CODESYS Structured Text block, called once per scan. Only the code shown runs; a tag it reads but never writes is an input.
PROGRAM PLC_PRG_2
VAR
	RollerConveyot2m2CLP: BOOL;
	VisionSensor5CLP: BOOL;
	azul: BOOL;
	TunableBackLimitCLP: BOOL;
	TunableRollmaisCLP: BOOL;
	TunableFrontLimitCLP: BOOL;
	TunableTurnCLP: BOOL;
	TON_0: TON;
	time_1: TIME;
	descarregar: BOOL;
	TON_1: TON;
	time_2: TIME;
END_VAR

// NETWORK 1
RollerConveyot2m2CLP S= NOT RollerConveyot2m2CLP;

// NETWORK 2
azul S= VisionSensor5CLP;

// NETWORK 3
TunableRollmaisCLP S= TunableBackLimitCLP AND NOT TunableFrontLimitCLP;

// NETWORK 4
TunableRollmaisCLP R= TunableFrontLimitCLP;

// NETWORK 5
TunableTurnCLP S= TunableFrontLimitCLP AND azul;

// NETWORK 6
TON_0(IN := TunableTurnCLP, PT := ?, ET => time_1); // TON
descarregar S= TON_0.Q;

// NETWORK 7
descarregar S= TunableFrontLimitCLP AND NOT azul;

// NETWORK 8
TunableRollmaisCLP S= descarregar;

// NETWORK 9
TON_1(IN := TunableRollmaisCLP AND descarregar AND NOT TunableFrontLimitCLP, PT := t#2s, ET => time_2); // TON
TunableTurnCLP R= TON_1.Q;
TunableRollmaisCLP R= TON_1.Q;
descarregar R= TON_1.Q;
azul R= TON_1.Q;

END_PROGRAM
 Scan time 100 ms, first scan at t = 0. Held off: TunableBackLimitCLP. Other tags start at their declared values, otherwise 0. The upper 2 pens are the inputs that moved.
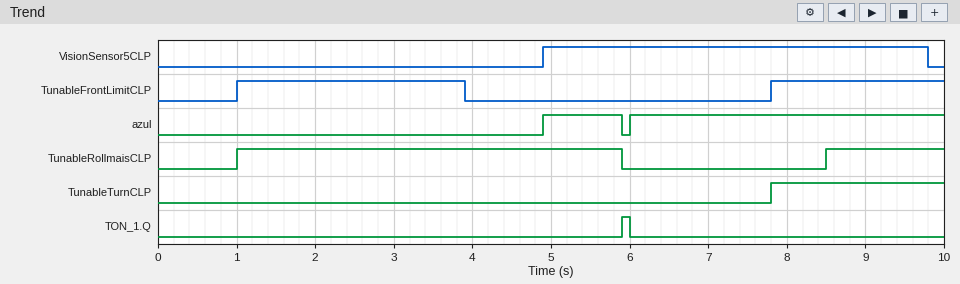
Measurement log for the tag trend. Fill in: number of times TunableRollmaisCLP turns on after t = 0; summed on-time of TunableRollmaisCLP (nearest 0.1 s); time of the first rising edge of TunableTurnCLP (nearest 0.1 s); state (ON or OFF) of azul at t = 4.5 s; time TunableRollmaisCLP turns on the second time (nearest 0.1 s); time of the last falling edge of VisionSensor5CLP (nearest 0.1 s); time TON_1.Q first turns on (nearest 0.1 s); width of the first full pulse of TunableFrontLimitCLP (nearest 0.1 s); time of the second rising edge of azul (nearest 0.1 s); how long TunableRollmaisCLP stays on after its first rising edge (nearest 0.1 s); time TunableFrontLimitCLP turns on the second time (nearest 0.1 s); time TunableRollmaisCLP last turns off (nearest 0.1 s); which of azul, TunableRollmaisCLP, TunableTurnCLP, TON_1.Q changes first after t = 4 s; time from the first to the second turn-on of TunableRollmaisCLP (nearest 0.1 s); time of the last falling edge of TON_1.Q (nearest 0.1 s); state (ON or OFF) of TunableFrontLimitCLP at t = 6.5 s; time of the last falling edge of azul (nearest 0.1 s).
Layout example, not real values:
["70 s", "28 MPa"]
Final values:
["2", "6.4 s", "7.8 s", "OFF", "8.5 s", "9.8 s", "5.9 s", "2.9 s", "6.0 s", "4.9 s", "7.8 s", "5.9 s", "azul", "7.5 s", "6.0 s", "OFF", "5.9 s"]
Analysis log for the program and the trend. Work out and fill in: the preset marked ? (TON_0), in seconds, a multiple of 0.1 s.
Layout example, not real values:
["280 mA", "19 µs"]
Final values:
["0.7 s"]
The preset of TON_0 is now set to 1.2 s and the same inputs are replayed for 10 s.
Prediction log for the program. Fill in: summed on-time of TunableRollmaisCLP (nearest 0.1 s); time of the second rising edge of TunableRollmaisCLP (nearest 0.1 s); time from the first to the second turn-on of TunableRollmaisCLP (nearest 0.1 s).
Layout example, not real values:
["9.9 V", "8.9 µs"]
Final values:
["5.9 s", "9.0 s", "8.0 s"]
